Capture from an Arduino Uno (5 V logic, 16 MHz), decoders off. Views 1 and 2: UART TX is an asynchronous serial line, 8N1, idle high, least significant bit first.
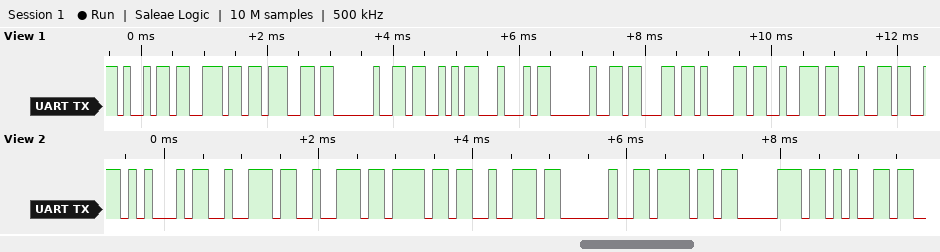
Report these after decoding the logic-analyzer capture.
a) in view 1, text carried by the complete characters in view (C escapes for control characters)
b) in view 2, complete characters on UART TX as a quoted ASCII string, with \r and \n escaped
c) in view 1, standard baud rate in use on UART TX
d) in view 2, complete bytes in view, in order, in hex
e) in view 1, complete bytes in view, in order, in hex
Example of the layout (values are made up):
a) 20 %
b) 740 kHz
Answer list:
a) "ing SD card"
b) "Error ope"
c) 9600 baud
d) 45 72 72 6F 72 20 6F 70 65
e) 69 6E 67 20 53 44 20 63 61 72 64
